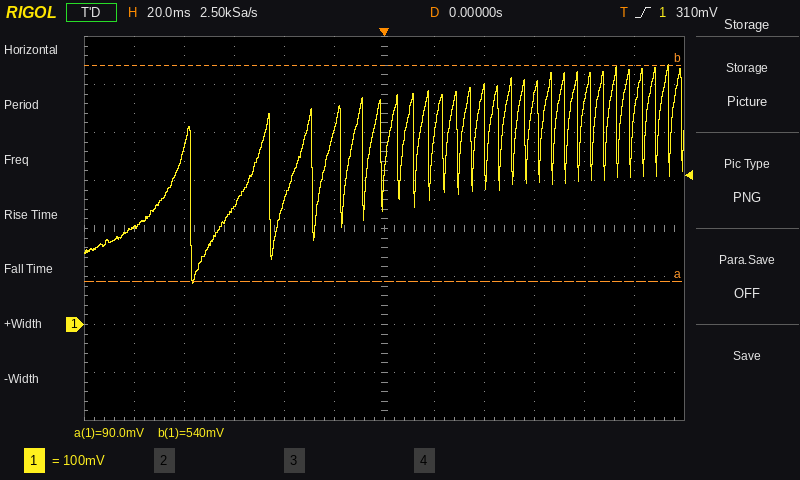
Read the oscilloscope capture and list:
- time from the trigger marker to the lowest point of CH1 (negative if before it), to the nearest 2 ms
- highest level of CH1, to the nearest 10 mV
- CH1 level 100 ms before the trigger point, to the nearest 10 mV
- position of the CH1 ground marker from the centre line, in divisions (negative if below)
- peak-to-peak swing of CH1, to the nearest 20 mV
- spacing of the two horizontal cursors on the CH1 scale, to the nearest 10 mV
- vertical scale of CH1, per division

-76 ms
540 mV
200 mV
-2.0 div
460 mV
450 mV
100 mV
